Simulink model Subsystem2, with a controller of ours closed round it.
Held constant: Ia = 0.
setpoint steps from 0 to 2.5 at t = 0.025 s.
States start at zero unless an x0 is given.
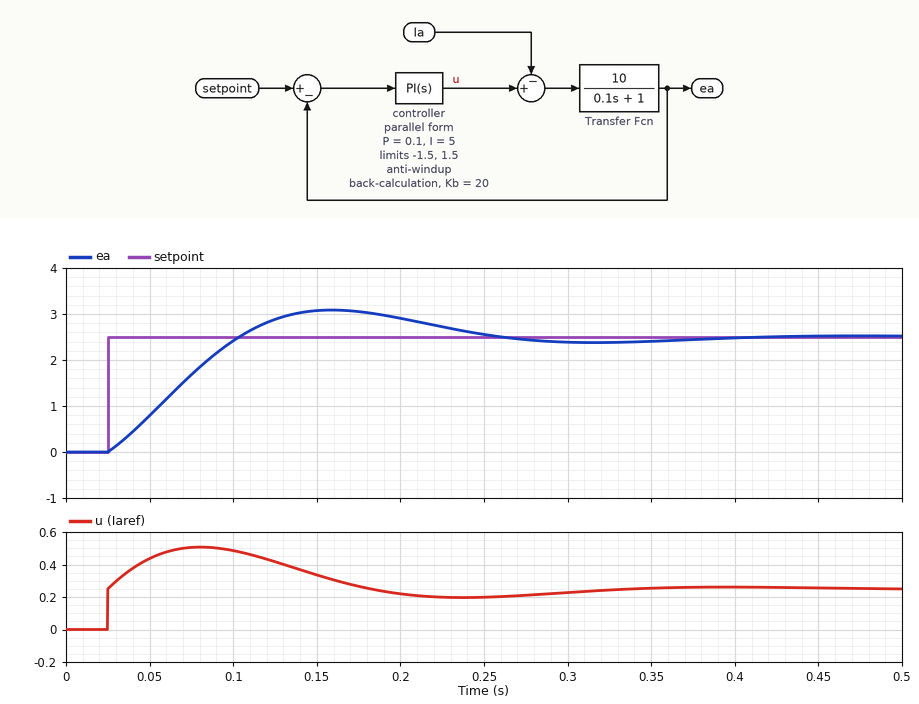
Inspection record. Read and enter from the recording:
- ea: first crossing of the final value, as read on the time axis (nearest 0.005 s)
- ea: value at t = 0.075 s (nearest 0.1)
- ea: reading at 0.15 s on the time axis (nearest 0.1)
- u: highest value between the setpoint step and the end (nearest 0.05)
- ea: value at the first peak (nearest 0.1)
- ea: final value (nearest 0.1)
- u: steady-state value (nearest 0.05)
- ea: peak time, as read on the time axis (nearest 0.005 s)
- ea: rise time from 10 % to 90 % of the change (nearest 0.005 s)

0.105 s
1.7
3.1
0.50
3.1
2.5
0.25
0.160 s
0.060 s
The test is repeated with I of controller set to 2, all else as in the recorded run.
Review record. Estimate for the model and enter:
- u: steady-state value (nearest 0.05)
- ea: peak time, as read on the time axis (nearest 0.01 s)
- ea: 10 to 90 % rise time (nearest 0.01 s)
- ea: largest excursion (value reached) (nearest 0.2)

0.25
0.26 s
0.11 s
2.6
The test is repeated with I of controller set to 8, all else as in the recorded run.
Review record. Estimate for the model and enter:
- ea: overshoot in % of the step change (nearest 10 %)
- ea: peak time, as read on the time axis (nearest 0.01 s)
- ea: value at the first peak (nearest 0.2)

30 %
0.13 s
3.4
